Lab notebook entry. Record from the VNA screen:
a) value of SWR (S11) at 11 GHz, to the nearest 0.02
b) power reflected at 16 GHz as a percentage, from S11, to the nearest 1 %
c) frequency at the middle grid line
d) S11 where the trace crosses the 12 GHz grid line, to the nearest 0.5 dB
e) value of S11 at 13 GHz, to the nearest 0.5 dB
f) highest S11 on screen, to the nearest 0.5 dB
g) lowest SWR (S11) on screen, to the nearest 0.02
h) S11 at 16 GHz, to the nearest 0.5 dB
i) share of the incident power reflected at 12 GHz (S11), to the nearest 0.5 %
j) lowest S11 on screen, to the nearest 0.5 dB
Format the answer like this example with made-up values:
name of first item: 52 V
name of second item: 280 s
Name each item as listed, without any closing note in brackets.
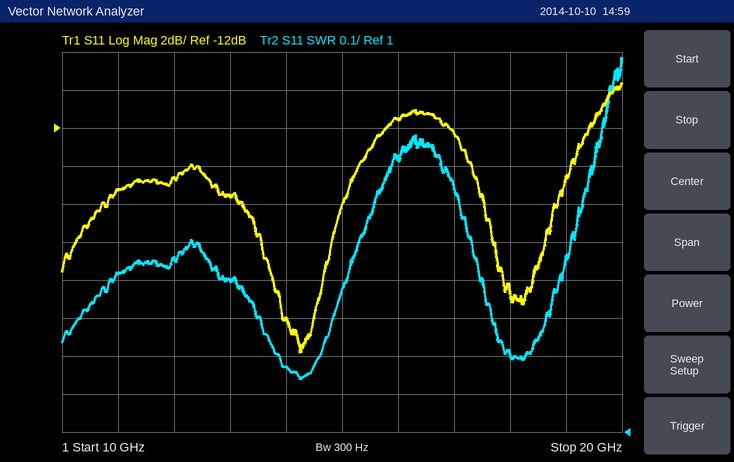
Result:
value of SWR (S11) at 11 GHz, to the nearest 0.02: 1.42
power reflected at 16 GHz as a percentage, from S11, to the nearest 1 %: 7 %
frequency at the middle grid line: 15 GHz
S11 where the trace crosses the 12 GHz grid line, to the nearest 0.5 dB: -14.5 dB
value of S11 at 13 GHz, to the nearest 0.5 dB: -15.5 dB
highest S11 on screen, to the nearest 0.5 dB: -9.5 dB
lowest SWR (S11) on screen, to the nearest 0.02: 1.14
S11 at 16 GHz, to the nearest 0.5 dB: -11.5 dB
share of the incident power reflected at 12 GHz (S11), to the nearest 0.5 %: 3.5 %
lowest S11 on screen, to the nearest 0.5 dB: -24.0 dB
